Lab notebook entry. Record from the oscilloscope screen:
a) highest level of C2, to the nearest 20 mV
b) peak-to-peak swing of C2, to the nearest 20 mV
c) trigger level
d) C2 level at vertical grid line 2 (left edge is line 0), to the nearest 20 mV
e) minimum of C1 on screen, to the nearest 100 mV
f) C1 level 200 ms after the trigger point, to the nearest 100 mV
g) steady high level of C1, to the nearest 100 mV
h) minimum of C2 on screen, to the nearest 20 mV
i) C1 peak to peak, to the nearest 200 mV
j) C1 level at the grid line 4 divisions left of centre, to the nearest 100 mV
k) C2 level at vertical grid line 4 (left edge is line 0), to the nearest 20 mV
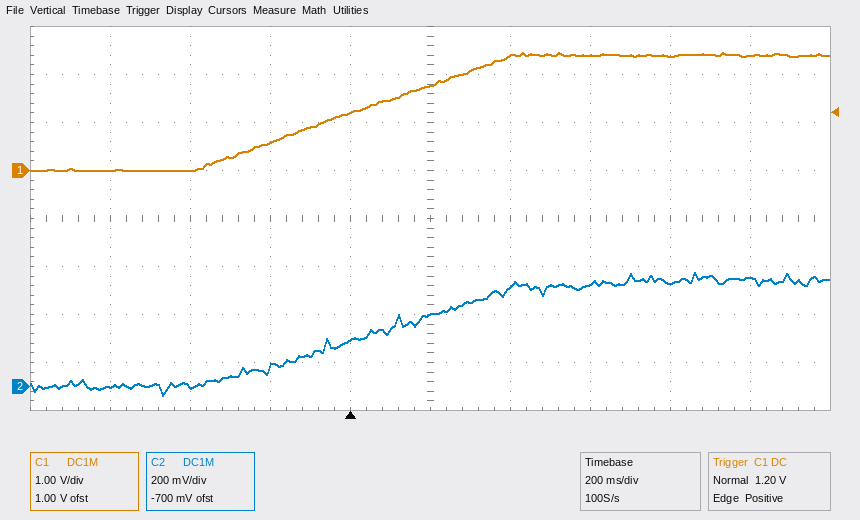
480 mV
520 mV
1.20 V
0 mV
0.0 V
1.8 V
2.4 V
-40 mV
2.4 V
0.0 V
200 mV
